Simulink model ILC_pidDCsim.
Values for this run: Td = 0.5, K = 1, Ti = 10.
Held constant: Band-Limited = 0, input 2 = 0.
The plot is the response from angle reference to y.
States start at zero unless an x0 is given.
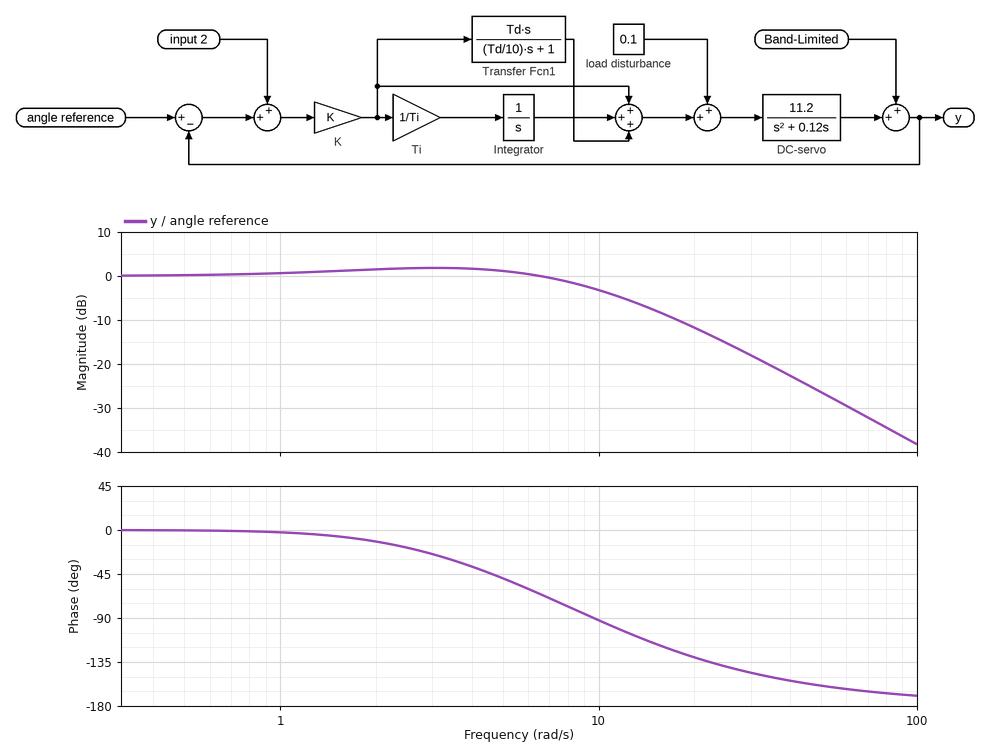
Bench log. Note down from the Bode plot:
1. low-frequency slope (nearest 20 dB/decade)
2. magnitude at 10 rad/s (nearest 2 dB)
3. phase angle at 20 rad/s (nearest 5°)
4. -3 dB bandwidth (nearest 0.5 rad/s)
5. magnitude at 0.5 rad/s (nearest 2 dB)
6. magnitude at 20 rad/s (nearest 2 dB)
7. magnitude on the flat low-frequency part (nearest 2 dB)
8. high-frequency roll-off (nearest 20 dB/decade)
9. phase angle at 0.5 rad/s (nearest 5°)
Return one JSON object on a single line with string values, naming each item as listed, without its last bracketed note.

{"low-frequency slope": "0 dB/decade", "magnitude at 10 rad/s": "-4 dB", "phase angle at 20 rad/s": "-130°", "-3 dB bandwidth": "9.5 rad/s", "magnitude at 0.5 rad/s": "0 dB", "magnitude at 20 rad/s": "-12 dB", "magnitude on the flat low-frequency part": "0 dB", "high-frequency roll-off": "-40 dB/decade", "phase angle at 0.5 rad/s": "0°"}
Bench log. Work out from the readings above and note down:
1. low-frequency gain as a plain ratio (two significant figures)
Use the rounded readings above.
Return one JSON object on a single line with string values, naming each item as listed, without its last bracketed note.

{"low-frequency gain as a plain ratio": "1.0"}
